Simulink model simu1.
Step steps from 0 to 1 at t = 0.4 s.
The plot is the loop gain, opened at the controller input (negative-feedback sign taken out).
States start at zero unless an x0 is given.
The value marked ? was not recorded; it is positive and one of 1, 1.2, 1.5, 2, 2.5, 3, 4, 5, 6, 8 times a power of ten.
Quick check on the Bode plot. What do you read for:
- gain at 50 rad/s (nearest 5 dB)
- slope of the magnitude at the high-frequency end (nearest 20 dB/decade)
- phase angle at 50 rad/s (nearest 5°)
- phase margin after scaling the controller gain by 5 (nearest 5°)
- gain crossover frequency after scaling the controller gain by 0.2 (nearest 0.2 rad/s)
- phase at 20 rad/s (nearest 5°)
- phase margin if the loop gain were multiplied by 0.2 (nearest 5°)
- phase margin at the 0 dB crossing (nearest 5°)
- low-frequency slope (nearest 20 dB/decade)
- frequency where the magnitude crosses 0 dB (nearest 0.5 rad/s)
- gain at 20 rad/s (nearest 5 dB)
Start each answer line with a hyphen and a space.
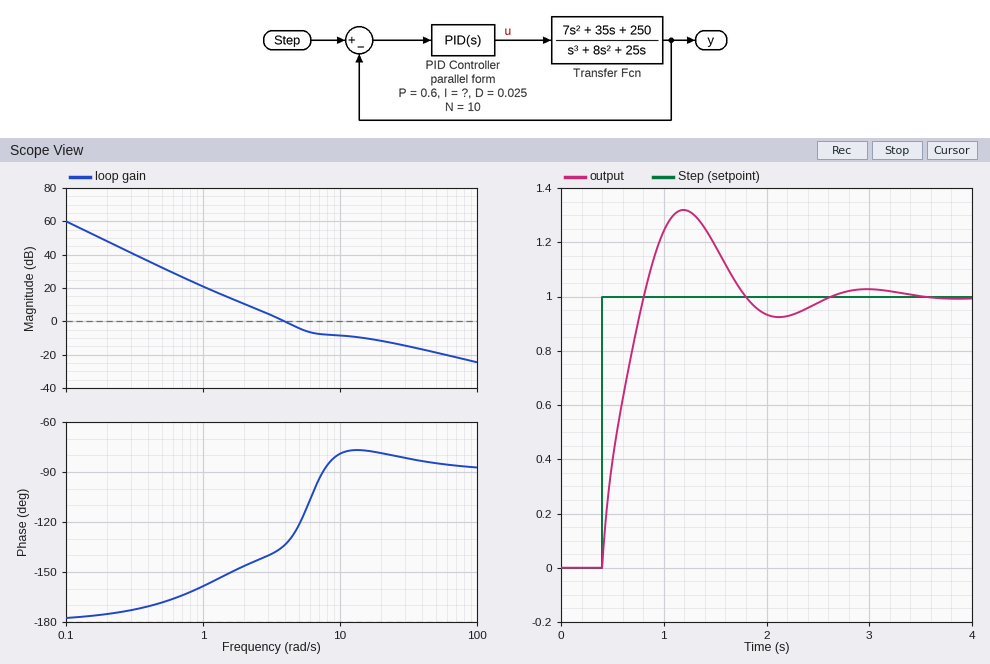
- -20 dB
- -20 dB/decade
- -85°
- 100°
- 1.6 rad/s
- -80°
- 30°
- 45°
- -40 dB/decade
- 4.0 rad/s
- -10 dB
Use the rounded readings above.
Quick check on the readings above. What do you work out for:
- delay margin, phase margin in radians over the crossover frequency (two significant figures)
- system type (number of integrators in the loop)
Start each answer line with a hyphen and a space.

- 0.20 s
- 2
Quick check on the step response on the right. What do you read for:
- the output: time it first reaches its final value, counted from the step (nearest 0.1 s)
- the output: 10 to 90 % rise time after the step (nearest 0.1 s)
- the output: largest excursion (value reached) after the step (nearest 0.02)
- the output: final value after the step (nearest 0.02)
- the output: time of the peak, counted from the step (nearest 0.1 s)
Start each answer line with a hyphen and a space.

- 0.4 s
- 0.3 s
- 1.32
- 1.00
- 0.8 s
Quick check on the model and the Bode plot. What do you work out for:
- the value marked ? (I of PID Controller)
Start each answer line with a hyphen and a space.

- 1
